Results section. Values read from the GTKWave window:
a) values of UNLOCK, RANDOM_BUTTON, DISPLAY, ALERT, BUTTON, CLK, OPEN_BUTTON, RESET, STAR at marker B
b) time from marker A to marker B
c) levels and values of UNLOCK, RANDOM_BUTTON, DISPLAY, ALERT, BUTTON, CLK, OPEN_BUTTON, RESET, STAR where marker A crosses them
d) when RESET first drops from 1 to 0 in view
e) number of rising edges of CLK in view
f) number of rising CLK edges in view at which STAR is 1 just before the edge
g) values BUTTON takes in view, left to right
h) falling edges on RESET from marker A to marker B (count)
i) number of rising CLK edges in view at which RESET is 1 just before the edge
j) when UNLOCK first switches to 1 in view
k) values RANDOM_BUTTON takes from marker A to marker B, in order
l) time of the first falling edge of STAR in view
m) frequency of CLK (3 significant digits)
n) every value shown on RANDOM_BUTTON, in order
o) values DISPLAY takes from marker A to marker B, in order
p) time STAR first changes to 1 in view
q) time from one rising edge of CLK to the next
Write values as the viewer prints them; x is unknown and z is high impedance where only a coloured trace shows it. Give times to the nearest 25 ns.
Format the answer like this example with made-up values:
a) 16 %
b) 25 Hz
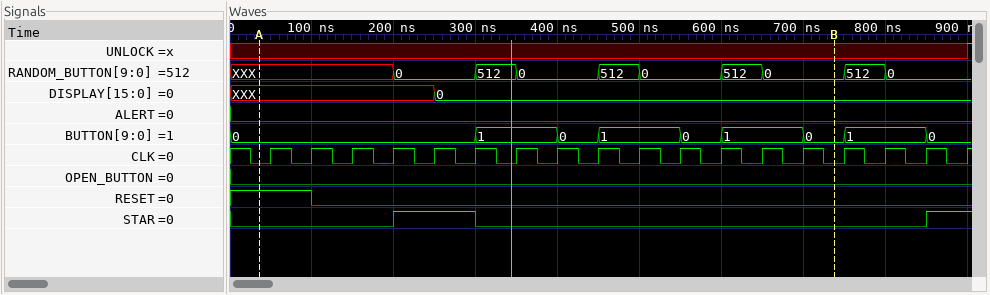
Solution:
a) UNLOCK=x, RANDOM_BUTTON=0, DISPLAY=0, ALERT=0, BUTTON=0, CLK=0, OPEN_BUTTON=0, RESET=0, STAR=0
b) 700 ns
c) UNLOCK=x, RANDOM_BUTTON=XXX, DISPLAY=XXX, ALERT=0, BUTTON=0, CLK=0, OPEN_BUTTON=0, RESET=1, STAR=0
d) 100 ns
e) 18
f) 3
g) 0, 1, 0, 1, 0, 1, 0, 1, 0
h) 1
i) 2
j) 900 ns
k) XXX, 0, 512, 0, 512, 0, 512, 0
l) 300 ns
m) 20.0 MHz
n) XXX, 0, 512, 0, 512, 0, 512, 0, 512, 0
o) XXX, 0
p) 200 ns
q) 50 ns
